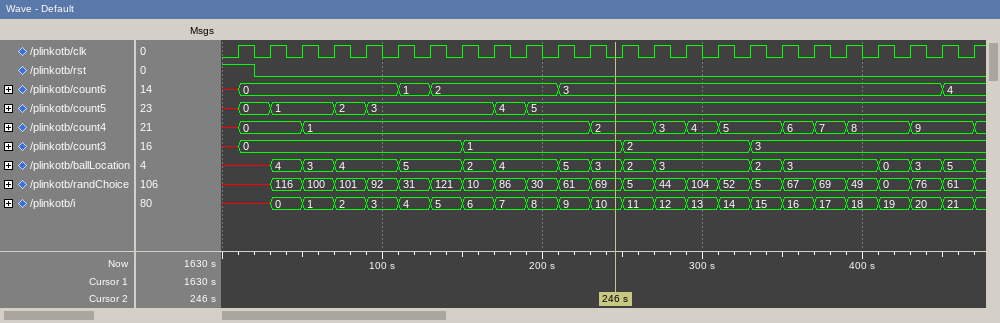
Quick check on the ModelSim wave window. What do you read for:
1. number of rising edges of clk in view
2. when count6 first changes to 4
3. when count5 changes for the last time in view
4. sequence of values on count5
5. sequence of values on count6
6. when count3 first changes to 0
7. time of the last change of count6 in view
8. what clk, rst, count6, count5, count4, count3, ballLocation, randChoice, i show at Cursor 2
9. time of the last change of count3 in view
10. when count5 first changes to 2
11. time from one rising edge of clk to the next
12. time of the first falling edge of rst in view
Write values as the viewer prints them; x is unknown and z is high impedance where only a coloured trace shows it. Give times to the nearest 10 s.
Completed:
24
450 s
190 s
x, 0, 1, 2, 3, 4, 5
x, 0, 1, 2, 3, 4
10 s
450 s
clk=0, rst=0, count6=3, count5=5, count4=2, count3=1, ballLocation=3, randChoice=69, i=10
330 s
70 s
20 s
20 s
